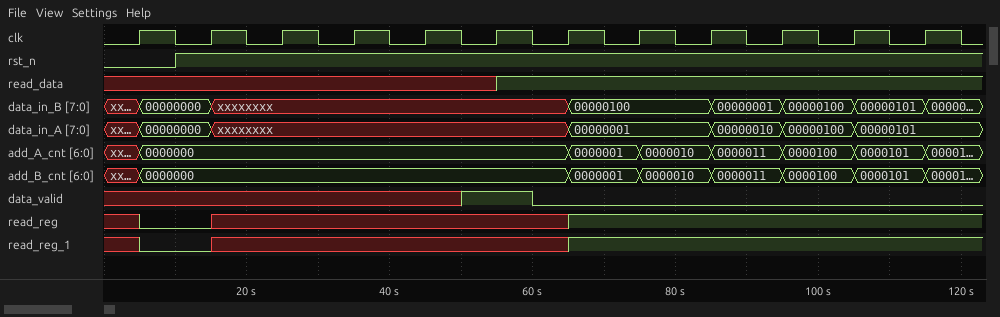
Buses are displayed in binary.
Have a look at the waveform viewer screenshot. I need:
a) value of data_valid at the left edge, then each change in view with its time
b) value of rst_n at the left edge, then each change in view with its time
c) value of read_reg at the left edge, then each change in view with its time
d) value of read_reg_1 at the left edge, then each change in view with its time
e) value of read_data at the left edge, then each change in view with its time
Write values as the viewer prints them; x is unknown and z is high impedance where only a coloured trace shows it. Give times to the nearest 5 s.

x, 1 at 50 s, 0 at 60 s
0, 1 at 10 s
x, 0 at 5 s, x at 15 s, 1 at 65 s
x, 0 at 5 s, x at 15 s, 1 at 65 s
x, 1 at 55 s
